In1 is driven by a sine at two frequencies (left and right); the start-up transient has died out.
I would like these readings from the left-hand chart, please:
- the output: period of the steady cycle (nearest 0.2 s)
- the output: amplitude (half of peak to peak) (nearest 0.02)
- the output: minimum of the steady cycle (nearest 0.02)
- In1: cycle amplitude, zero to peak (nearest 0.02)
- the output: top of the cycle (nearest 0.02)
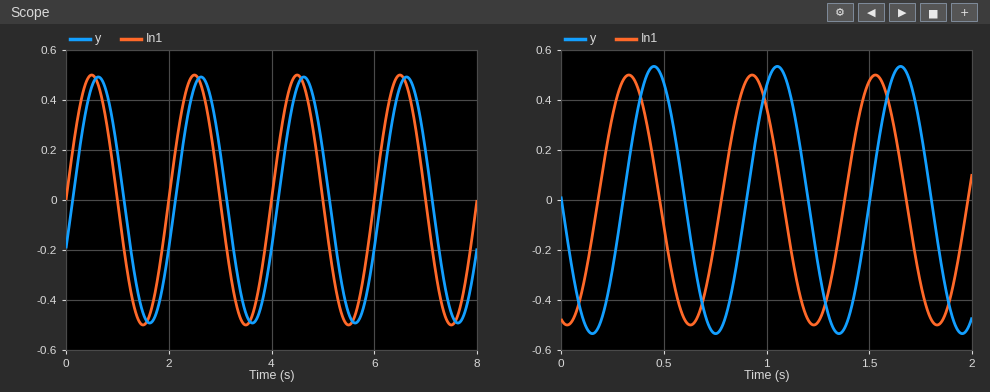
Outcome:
2.0 s
0.50
-0.50
0.50
0.50
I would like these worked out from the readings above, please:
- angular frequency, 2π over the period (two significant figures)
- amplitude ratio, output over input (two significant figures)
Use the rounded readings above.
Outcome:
3.1 rad/s
1.0
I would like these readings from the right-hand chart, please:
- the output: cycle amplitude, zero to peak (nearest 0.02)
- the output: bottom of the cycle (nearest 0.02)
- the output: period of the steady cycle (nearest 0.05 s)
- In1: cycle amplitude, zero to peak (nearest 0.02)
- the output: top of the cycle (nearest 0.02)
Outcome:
0.54
-0.54
0.60 s
0.50
0.54
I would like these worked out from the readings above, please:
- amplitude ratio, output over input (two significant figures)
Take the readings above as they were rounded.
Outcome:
1.1
